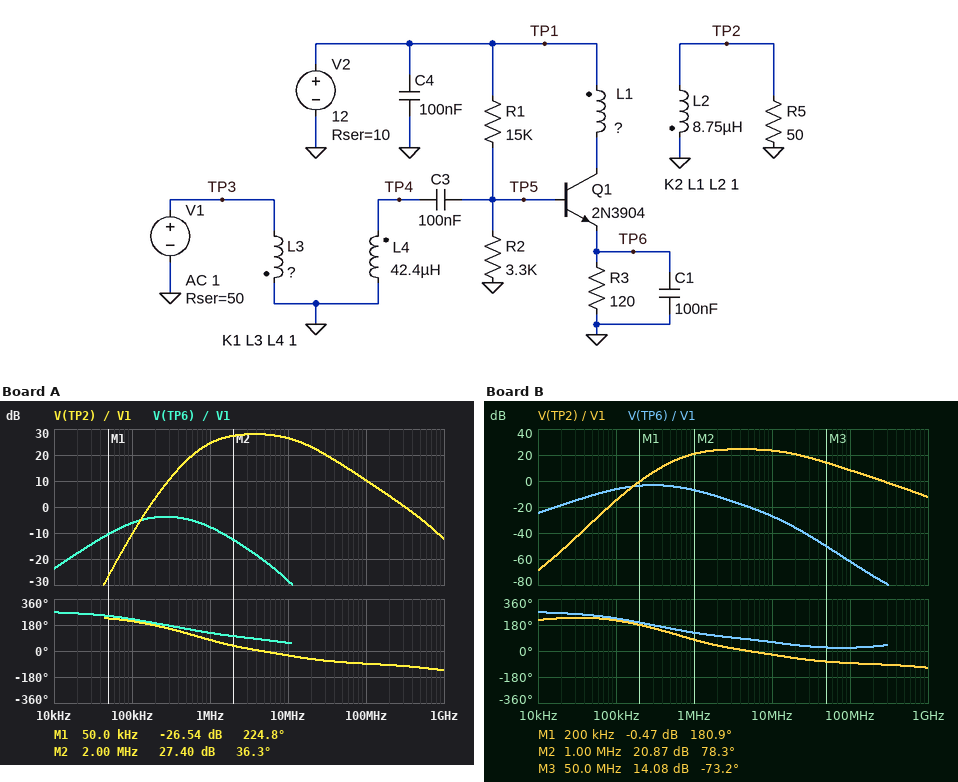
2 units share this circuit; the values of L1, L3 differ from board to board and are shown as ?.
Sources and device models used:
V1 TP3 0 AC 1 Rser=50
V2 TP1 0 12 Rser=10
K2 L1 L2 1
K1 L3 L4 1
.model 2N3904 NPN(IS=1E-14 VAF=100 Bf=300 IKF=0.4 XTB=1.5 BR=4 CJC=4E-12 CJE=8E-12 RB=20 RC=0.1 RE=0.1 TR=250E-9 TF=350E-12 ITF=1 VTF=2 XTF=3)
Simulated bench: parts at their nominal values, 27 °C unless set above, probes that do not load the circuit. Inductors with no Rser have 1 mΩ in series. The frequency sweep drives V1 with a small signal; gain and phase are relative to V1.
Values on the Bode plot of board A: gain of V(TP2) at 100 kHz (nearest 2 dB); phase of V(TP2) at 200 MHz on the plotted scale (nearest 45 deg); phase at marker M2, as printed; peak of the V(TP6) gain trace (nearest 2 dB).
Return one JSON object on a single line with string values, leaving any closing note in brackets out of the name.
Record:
{"gain of V(TP2) at 100 kHz": "-10 dB", "phase of V(TP2) at 200 MHz on the plotted scale": "-90 deg", "phase at marker M2, as printed": "36.3 deg", "peak of the V(TP6) gain trace": "-4 dB"}
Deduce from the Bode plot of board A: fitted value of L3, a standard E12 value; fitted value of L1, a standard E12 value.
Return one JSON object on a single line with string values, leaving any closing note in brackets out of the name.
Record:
{"fitted value of L3, a standard E12 value": "68 µH", "fitted value of L1, a standard E12 value": "27 µH"}
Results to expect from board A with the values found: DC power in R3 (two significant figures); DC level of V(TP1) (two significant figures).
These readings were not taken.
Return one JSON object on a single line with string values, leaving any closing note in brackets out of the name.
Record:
{"DC power in R3": "15 mW", "DC level of V(TP1)": "12 V"}
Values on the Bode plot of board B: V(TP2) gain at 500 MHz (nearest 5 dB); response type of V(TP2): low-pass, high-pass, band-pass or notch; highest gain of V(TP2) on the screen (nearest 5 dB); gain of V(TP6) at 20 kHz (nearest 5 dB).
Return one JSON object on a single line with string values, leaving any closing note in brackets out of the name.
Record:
{"V(TP2) gain at 500 MHz": "-5 dB", "response type of V(TP2): low-pass, high-pass, band-pass or notch": "band-pass", "highest gain of V(TP2) on the screen": "25 dB", "gain of V(TP6) at 20 kHz": "-20 dB"}
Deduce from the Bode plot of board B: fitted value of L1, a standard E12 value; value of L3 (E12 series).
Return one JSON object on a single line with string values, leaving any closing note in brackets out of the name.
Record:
{"fitted value of L1, a standard E12 value": "10 µH", "value of L3": "56 µH"}
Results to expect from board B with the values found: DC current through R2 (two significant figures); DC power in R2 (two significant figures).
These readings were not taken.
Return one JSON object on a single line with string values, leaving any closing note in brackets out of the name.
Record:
{"DC current through R2": "620 µA", "DC power in R2": "1.3 mW"}
